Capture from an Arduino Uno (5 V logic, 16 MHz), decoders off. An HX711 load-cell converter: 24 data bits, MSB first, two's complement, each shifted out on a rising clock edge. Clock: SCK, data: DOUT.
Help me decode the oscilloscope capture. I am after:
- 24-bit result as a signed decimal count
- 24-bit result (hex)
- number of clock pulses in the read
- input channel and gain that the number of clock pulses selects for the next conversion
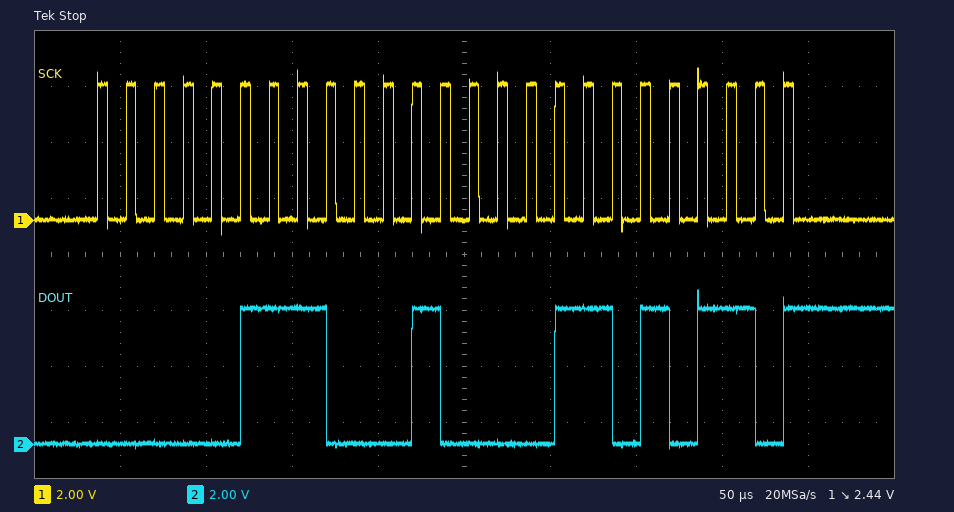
463062
0x0710D6
25
channel A, gain 128
